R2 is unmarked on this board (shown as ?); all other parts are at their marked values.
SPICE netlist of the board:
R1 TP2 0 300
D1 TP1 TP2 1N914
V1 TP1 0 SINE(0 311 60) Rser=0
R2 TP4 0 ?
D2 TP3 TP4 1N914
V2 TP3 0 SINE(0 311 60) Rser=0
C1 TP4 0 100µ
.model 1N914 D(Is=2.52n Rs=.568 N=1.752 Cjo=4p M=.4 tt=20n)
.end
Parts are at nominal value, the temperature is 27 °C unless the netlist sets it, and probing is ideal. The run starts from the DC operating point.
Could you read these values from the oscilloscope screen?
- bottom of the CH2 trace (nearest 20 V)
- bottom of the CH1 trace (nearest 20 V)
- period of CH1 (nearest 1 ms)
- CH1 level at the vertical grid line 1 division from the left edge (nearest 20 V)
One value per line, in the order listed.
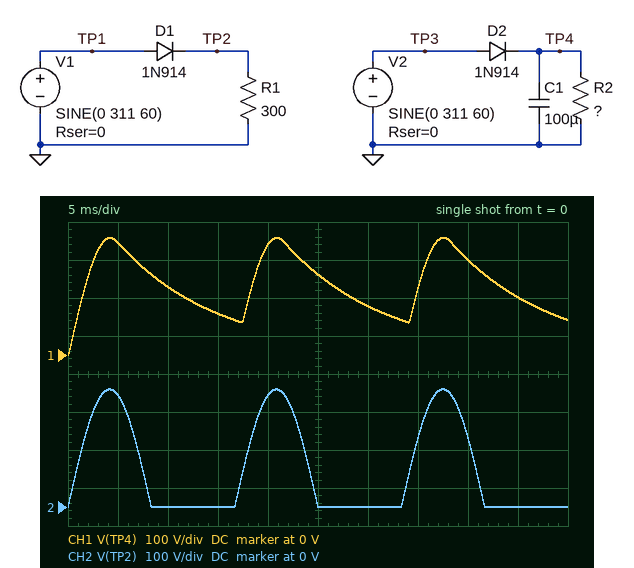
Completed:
0 V
0 V
17 ms
300 V
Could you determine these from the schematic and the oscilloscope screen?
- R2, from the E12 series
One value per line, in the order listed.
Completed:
100 Ω
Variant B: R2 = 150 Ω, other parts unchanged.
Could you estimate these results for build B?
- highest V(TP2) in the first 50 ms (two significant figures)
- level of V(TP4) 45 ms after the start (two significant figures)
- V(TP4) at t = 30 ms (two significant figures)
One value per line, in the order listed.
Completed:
310 V
190 V
170 V
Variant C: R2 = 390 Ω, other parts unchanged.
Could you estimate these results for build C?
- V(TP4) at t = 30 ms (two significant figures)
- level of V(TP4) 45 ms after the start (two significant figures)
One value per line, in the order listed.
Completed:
250 V
260 V
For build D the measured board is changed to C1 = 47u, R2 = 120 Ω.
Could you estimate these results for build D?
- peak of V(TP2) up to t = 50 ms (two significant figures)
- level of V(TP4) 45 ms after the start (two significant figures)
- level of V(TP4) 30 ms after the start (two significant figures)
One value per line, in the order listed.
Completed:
310 V
91 V
68 V
